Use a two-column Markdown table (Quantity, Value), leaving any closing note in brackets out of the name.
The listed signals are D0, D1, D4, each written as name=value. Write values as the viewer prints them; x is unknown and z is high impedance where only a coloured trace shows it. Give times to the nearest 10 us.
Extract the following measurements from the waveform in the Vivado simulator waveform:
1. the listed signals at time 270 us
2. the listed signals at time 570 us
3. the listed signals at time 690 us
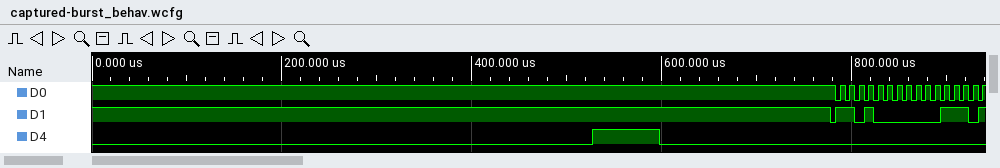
| Quantity | Value |
|---|---|
| the listed signals at time 270 us | D0=1, D1=1, D4=0 |
| the listed signals at time 570 us | D0=1, D1=1, D4=1 |
| the listed signals at time 690 us | D0=1, D1=1, D4=0 |
